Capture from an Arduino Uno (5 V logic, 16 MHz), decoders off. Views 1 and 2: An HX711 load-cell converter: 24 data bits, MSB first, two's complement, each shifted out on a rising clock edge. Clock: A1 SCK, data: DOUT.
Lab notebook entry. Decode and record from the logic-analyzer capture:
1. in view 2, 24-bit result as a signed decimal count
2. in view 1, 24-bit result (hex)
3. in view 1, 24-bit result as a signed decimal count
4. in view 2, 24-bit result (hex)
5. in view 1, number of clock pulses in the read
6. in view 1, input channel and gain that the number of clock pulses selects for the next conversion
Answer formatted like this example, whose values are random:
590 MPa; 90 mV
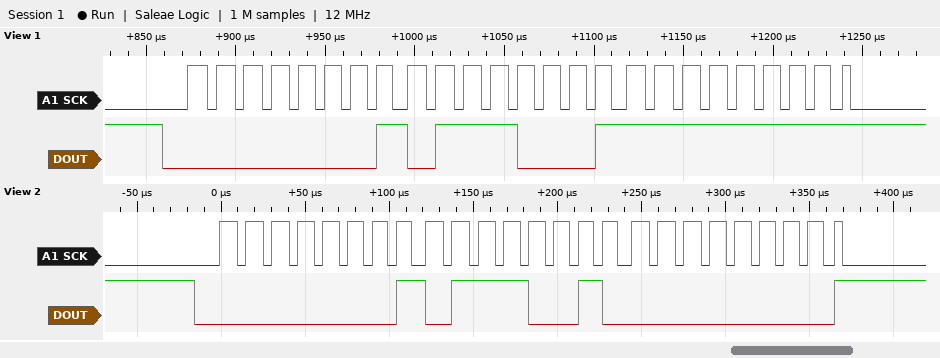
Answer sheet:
94720; 0x0171FF; 94719; 0x017200; 25; channel A, gain 128
